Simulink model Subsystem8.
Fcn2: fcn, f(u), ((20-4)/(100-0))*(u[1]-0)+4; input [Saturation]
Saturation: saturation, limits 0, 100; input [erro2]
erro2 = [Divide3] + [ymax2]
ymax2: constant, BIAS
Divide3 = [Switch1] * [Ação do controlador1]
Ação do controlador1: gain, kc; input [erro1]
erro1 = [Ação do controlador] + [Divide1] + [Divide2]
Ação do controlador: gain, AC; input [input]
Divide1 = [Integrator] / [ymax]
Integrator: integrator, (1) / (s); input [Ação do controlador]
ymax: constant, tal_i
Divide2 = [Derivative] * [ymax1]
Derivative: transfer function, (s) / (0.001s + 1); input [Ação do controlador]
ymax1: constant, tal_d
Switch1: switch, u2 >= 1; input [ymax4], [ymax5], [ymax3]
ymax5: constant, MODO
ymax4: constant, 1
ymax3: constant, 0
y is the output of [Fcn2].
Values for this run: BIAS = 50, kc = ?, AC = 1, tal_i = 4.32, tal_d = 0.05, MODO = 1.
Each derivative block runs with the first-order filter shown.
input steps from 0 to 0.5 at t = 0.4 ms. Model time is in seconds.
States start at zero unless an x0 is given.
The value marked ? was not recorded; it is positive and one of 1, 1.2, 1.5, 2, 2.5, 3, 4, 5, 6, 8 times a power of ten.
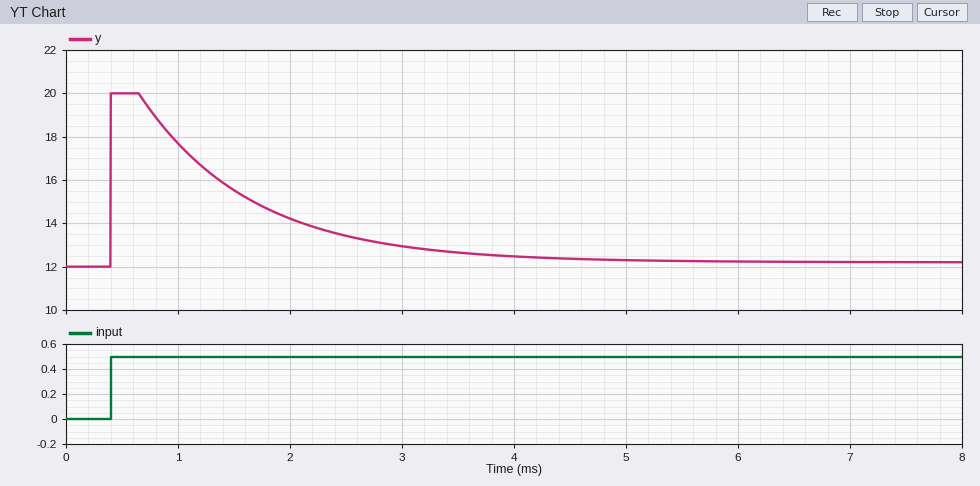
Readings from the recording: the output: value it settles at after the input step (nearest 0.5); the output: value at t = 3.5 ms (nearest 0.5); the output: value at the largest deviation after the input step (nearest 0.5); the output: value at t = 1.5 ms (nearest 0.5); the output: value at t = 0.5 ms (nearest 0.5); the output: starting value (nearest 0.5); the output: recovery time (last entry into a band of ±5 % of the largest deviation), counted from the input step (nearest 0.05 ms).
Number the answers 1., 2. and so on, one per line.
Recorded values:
1. 12.0
2. 12.5
3. 20.0
4. 15.5
5. 20.0
6. 12.0
7. 3.20 ms
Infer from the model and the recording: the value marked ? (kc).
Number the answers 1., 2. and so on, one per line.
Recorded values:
1. 2.5
